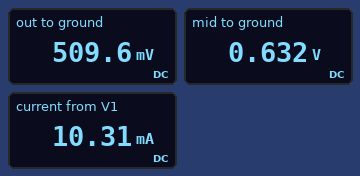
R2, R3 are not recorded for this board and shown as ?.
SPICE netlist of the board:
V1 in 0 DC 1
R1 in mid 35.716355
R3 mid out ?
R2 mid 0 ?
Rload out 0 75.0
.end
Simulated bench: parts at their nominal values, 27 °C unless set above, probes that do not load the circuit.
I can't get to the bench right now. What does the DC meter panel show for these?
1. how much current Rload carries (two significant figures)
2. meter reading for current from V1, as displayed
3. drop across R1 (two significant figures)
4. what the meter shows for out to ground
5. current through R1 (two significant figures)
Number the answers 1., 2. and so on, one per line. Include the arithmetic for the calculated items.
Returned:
1. (509.6 mV) / 75 Ω = 6.8 mA
2. 10.31 mA
3. 1 V - 632 mV = 370 mV
4. 509.6 mV
5. (1 V - 632 mV) / 35.72 Ω = 10 mA
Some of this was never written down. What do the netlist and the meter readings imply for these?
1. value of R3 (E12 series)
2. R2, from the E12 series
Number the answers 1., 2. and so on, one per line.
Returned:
1. 18 Ω
2. 180 Ω
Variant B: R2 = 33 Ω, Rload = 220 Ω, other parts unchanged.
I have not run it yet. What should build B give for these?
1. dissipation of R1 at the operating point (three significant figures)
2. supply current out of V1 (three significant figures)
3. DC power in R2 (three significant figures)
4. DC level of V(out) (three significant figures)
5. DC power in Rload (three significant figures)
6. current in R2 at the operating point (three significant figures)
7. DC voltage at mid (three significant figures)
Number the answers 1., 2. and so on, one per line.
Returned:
1. 8.53 mW
2. 15.5 mA
3. 6.08 mW
4. 414 mV
5. 779 µW
6. 13.6 mA
7. 448 mV
